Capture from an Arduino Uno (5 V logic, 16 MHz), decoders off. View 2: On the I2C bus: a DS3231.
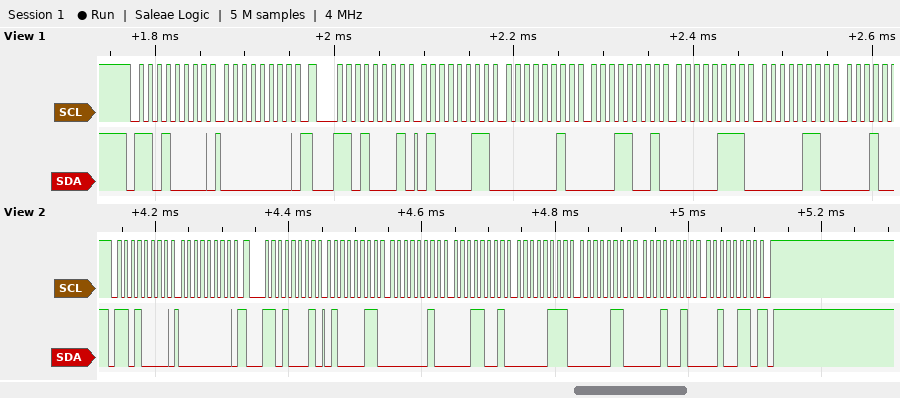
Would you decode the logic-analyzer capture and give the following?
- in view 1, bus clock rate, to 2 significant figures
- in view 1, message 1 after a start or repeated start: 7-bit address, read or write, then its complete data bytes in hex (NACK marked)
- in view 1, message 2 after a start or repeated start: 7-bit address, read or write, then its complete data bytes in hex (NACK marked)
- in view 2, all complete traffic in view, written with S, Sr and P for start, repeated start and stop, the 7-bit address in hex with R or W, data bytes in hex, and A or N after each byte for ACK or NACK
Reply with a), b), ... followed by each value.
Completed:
a) 100 kHz
b) 0x68 write: 00
c) 0x68 read: 43 02 19 07 06
d) S 68W A 00 A Sr 68R A 43 A 02 A 19 A 07 A 06 A 12 A 26 N P
